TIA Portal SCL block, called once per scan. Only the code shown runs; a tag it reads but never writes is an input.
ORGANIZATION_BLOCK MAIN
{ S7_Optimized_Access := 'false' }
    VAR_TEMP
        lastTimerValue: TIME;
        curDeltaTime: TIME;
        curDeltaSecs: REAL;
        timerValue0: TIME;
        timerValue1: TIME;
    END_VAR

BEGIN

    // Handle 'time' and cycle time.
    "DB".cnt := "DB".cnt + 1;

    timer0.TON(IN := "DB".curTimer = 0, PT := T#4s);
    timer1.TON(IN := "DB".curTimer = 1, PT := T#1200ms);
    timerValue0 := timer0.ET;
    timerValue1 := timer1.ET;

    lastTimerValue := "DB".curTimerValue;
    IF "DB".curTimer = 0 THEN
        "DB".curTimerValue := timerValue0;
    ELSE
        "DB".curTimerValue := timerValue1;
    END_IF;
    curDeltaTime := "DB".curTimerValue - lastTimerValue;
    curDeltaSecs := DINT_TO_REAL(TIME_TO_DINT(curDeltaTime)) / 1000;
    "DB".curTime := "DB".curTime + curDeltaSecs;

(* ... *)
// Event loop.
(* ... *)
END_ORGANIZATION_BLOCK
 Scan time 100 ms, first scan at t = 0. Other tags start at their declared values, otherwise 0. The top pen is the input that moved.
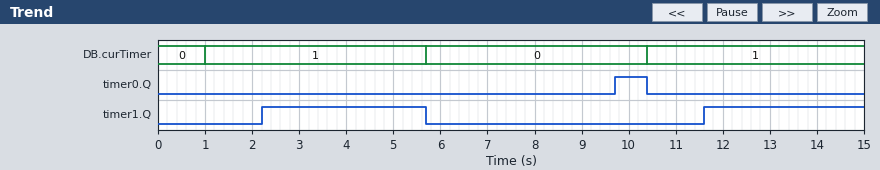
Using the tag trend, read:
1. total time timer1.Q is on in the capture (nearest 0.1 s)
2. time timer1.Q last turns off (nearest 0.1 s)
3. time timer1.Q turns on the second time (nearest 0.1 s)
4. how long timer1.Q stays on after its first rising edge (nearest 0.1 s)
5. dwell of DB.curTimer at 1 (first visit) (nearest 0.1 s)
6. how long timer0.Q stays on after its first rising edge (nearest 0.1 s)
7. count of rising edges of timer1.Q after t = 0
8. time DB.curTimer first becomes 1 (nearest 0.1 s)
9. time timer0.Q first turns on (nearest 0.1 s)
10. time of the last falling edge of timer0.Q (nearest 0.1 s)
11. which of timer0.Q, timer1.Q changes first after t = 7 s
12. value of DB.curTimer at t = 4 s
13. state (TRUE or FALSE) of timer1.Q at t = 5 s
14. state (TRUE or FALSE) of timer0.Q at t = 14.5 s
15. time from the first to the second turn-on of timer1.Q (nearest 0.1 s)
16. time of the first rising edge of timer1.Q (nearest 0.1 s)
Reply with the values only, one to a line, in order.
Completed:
6.9 s
5.7 s
11.6 s
3.5 s
4.7 s
0.7 s
2
1.0 s
9.7 s
10.4 s
timer0.Q
1
TRUE
FALSE
9.4 s
2.2 s
